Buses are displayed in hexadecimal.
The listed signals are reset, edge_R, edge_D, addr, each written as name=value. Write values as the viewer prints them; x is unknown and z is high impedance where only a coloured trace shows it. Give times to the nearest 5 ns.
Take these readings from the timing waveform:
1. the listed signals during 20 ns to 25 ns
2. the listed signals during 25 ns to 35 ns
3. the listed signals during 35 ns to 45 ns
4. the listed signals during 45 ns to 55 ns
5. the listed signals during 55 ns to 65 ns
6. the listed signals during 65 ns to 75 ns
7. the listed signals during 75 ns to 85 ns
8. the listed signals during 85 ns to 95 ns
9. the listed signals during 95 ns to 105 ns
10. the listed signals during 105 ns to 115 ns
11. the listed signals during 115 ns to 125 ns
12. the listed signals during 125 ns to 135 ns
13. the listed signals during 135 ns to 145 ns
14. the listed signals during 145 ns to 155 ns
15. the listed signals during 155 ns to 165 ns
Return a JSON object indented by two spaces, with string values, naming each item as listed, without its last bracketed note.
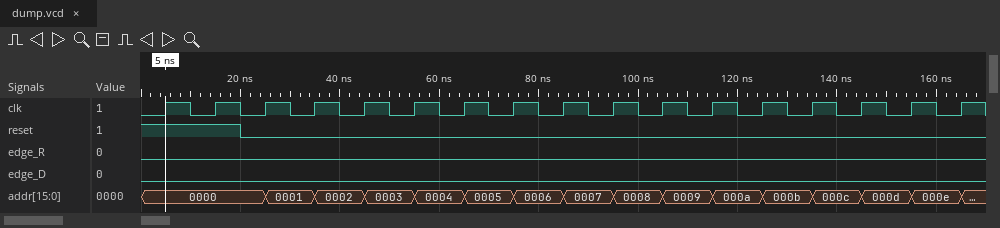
{
  "the listed signals during 20 ns to 25 ns": "reset=0, edge_R=0, edge_D=0, addr=0000",
  "the listed signals during 25 ns to 35 ns": "reset=0, edge_R=0, edge_D=0, addr=0001",
  "the listed signals during 35 ns to 45 ns": "reset=0, edge_R=0, edge_D=0, addr=0002",
  "the listed signals during 45 ns to 55 ns": "reset=0, edge_R=0, edge_D=0, addr=0003",
  "the listed signals during 55 ns to 65 ns": "reset=0, edge_R=0, edge_D=0, addr=0004",
  "the listed signals during 65 ns to 75 ns": "reset=0, edge_R=0, edge_D=0, addr=0005",
  "the listed signals during 75 ns to 85 ns": "reset=0, edge_R=0, edge_D=0, addr=0006",
  "the listed signals during 85 ns to 95 ns": "reset=0, edge_R=0, edge_D=0, addr=0007",
  "the listed signals during 95 ns to 105 ns": "reset=0, edge_R=0, edge_D=0, addr=0008",
  "the listed signals during 105 ns to 115 ns": "reset=0, edge_R=0, edge_D=0, addr=0009",
  "the listed signals during 115 ns to 125 ns": "reset=0, edge_R=0, edge_D=0, addr=000a",
  "the listed signals during 125 ns to 135 ns": "reset=0, edge_R=0, edge_D=0, addr=000b",
  "the listed signals during 135 ns to 145 ns": "reset=0, edge_R=0, edge_D=0, addr=000c",
  "the listed signals during 145 ns to 155 ns": "reset=0, edge_R=0, edge_D=0, addr=000d",
  "the listed signals during 155 ns to 165 ns": "reset=0, edge_R=0, edge_D=0, addr=000e"
}
